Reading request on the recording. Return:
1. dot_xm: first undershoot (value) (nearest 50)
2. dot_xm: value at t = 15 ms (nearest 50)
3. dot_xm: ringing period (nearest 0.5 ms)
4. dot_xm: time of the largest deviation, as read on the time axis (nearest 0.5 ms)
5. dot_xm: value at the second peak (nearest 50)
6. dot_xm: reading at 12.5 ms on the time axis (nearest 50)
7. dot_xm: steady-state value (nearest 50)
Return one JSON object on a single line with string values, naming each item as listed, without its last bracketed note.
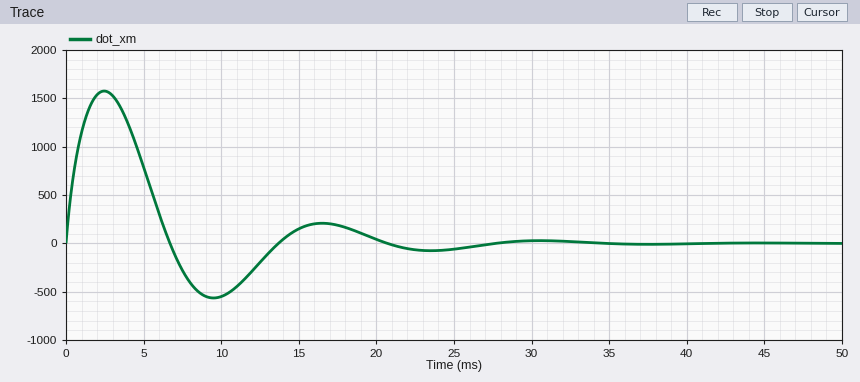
{"dot_xm: first undershoot (value)": "-550", "dot_xm: value at t = 15 ms": "150", "dot_xm: ringing period": "14.0 ms", "dot_xm: time of the largest deviation, as read on the time axis": "2.5 ms", "dot_xm: value at the second peak": "200", "dot_xm: reading at 12.5 ms on the time axis": "-200", "dot_xm: steady-state value": "0"}
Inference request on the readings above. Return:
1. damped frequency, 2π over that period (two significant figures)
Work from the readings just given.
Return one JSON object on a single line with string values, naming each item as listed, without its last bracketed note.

{"damped frequency, 2π over that period": "0.45 rad/ms"}
